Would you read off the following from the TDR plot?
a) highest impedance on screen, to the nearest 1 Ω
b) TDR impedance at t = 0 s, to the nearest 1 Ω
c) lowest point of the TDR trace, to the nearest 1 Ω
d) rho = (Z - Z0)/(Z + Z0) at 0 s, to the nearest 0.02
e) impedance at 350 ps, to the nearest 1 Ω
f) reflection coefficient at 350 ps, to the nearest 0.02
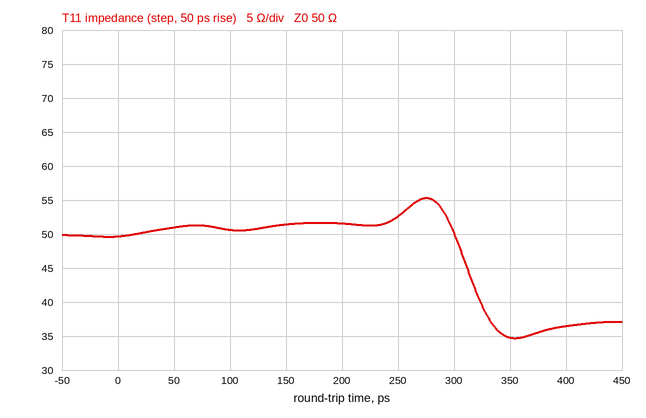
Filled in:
55 Ω
50 Ω
35 Ω
0.00
35 Ω
-0.18
